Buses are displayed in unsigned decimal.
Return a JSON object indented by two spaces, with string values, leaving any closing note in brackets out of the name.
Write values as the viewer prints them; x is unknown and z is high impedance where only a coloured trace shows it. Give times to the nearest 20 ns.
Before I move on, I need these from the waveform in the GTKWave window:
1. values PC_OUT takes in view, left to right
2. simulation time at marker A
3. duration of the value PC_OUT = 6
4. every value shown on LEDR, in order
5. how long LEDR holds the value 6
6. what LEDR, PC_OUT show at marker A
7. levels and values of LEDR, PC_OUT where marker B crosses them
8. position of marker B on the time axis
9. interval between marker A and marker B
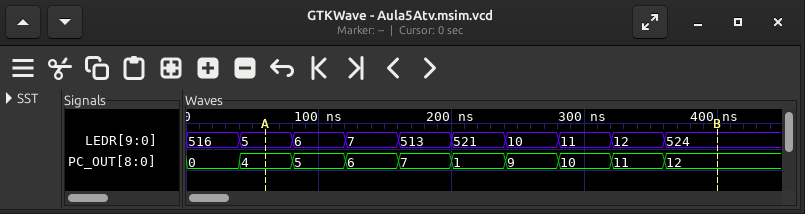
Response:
{
  "values PC_OUT takes in view, left to right": "0, 4, 5, 6, 7, 1, 9, 10, 11, 12",
  "simulation time at marker A": "60 ns",
  "duration of the value PC_OUT = 6": "40 ns",
  "every value shown on LEDR, in order": "516, 5, 6, 7, 513, 521, 10, 11, 12, 524",
  "how long LEDR holds the value 6": "40 ns",
  "what LEDR, PC_OUT show at marker A": "LEDR=5, PC_OUT=4",
  "levels and values of LEDR, PC_OUT where marker B crosses them": "LEDR=524, PC_OUT=12",
  "position of marker B on the time axis": "400 ns",
  "interval between marker A and marker B": "340 ns"
}
